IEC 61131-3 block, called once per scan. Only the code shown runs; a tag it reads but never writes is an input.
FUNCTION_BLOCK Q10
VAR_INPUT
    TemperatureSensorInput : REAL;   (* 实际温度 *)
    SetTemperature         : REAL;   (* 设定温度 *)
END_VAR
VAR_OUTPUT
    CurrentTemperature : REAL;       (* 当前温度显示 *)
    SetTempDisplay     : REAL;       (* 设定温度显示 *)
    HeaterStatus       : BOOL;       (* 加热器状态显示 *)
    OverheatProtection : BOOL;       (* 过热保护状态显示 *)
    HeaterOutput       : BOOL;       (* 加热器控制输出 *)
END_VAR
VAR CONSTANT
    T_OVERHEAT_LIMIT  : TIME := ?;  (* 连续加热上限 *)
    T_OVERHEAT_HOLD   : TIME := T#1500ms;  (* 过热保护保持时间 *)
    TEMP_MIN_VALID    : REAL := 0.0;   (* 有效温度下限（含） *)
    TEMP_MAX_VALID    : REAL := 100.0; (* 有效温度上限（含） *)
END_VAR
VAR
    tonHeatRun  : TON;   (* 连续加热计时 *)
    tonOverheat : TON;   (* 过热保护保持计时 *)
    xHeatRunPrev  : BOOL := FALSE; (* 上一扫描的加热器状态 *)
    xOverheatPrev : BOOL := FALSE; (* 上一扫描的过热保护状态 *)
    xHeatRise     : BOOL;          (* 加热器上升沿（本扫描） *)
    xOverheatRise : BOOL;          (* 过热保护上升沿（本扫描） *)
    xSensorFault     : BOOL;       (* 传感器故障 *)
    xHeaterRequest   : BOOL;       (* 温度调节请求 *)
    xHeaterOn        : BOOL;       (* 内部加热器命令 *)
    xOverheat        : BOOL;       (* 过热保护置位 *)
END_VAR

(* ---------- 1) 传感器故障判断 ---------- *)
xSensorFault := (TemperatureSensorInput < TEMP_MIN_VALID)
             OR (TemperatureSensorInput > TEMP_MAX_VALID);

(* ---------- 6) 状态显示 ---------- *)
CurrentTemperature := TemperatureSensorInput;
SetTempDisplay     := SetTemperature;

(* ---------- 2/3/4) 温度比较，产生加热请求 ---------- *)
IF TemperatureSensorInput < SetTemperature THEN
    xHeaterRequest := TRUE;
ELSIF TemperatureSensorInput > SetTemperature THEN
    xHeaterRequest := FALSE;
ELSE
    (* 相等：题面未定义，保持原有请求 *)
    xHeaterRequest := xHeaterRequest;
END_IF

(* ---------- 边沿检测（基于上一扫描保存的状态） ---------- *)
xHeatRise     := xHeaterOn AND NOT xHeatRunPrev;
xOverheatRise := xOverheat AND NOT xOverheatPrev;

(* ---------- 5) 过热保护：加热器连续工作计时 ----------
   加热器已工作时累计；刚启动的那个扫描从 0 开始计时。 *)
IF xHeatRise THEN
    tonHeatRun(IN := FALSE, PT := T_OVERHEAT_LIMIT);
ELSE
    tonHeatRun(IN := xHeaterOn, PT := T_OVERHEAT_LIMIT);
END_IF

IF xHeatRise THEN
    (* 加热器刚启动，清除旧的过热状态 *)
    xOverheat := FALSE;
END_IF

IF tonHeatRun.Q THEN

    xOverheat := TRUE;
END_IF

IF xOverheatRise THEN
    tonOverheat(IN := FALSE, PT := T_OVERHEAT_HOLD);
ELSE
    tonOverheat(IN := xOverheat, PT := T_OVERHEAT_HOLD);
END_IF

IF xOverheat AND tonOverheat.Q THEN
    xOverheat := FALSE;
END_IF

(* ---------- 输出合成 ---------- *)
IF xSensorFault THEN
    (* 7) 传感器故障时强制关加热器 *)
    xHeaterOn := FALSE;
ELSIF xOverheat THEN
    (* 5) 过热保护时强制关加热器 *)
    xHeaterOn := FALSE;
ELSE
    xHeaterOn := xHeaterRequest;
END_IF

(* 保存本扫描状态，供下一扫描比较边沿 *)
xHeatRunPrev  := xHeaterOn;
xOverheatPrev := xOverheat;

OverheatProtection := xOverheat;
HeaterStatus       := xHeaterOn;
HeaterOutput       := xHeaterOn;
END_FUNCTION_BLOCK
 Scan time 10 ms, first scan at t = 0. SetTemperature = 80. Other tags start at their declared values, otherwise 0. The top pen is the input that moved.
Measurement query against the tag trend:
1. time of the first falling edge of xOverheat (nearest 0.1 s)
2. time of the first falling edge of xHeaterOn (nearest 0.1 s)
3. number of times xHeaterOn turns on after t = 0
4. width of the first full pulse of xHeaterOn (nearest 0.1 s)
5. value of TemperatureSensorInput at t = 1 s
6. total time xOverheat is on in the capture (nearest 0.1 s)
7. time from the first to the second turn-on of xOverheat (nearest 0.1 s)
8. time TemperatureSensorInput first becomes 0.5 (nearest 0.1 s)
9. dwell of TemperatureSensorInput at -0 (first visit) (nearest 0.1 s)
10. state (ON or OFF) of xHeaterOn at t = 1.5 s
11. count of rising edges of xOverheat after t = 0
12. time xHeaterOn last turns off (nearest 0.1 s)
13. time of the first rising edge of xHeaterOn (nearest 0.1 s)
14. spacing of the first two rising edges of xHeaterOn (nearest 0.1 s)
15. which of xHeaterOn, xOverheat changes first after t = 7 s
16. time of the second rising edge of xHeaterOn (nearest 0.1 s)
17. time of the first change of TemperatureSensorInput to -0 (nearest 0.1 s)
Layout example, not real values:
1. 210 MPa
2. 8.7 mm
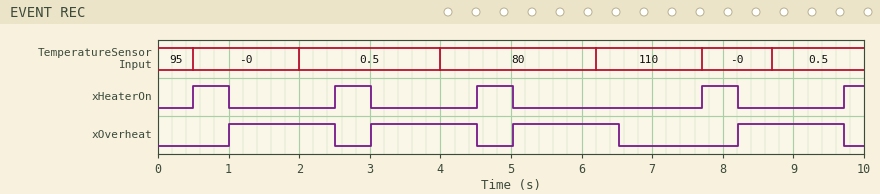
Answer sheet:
1. 2.5 s
2. 1.0 s
3. 5
4. 0.5 s
5. -0
6. 6.0 s
7. 2.0 s
8. 2.0 s
9. 1.5 s
10. OFF
11. 4
12. 8.2 s
13. 0.5 s
14. 2.0 s
15. xHeaterOn
16. 2.5 s
17. 0.5 s
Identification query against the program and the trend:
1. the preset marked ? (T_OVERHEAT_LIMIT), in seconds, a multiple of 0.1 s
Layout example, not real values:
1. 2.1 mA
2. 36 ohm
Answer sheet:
1. 0.5 s
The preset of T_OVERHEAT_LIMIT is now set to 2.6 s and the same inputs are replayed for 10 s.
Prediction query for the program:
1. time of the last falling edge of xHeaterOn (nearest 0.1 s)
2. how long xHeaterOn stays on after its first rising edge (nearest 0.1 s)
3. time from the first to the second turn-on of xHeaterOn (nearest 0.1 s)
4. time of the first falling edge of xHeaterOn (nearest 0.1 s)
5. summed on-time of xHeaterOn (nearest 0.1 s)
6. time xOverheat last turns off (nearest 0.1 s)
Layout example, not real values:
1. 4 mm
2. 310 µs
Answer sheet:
1. 6.2 s
2. 2.6 s
3. 4.1 s
4. 3.1 s
5. 6.5 s
6. 4.6 s
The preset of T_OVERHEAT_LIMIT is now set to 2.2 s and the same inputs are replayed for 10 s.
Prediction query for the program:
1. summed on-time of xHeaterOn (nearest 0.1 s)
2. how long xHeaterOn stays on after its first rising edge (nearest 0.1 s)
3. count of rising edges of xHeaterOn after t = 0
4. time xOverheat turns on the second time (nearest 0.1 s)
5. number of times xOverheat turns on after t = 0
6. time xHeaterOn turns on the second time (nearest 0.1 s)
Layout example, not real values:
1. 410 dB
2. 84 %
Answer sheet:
1. 6.4 s
2. 2.2 s
3. 3
4. 9.9 s
5. 2
6. 4.2 s
